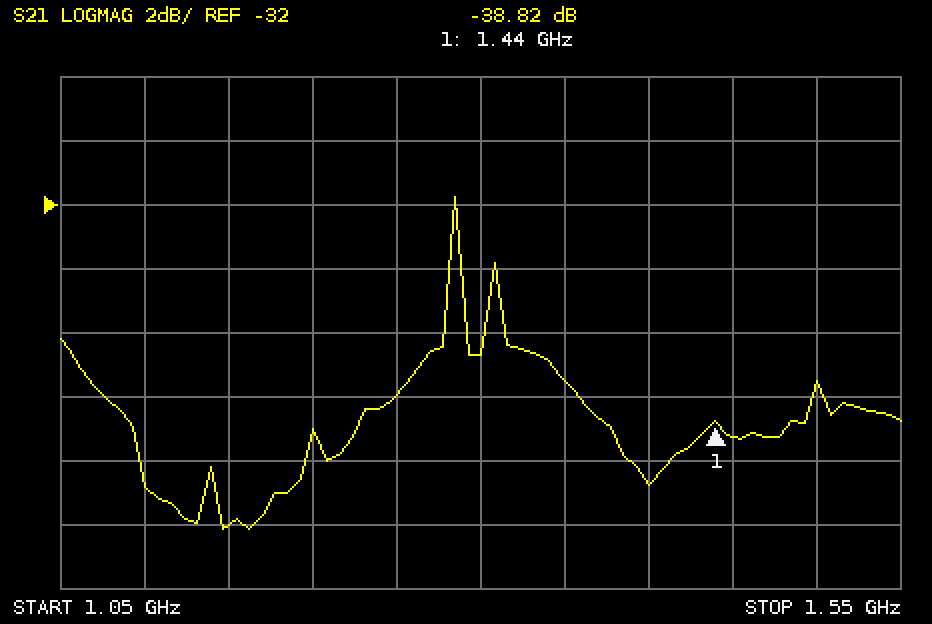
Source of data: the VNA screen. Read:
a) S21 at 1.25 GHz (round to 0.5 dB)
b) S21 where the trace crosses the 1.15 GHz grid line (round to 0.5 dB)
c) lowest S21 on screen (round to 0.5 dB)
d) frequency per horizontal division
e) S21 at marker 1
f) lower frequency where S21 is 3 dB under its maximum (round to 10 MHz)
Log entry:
-38.0 dB
-42.0 dB
-42.0 dB
50 MHz
-38.82 dB
1.28 GHz
